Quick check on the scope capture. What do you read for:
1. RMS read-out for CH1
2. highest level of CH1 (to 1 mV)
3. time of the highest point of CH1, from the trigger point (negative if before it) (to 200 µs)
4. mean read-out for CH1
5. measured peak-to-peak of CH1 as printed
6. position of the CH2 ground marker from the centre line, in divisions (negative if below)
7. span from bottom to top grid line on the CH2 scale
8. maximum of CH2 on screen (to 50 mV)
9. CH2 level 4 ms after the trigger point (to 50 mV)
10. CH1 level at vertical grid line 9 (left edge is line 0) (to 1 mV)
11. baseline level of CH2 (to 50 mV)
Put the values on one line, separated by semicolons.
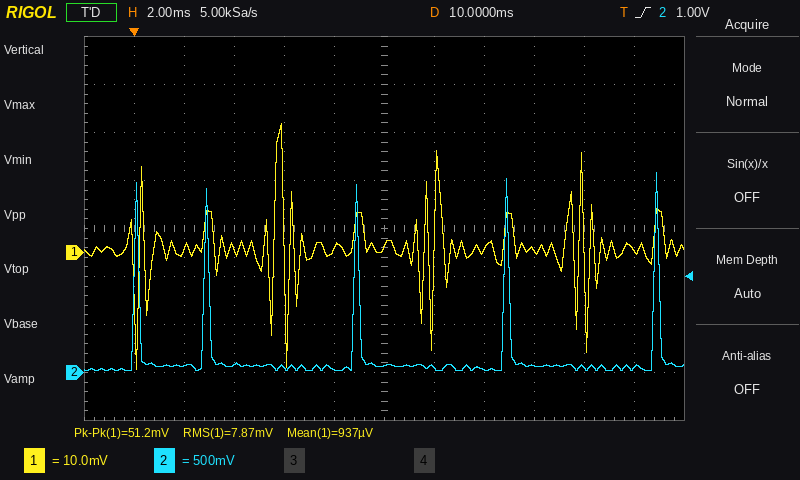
7.87 mV; 27 mV; +5.8 ms; 937 µV; 51.2 mV; -3.0 div; 4 V; 2.10 V; 100 mV; 0 mV; 50 mV
